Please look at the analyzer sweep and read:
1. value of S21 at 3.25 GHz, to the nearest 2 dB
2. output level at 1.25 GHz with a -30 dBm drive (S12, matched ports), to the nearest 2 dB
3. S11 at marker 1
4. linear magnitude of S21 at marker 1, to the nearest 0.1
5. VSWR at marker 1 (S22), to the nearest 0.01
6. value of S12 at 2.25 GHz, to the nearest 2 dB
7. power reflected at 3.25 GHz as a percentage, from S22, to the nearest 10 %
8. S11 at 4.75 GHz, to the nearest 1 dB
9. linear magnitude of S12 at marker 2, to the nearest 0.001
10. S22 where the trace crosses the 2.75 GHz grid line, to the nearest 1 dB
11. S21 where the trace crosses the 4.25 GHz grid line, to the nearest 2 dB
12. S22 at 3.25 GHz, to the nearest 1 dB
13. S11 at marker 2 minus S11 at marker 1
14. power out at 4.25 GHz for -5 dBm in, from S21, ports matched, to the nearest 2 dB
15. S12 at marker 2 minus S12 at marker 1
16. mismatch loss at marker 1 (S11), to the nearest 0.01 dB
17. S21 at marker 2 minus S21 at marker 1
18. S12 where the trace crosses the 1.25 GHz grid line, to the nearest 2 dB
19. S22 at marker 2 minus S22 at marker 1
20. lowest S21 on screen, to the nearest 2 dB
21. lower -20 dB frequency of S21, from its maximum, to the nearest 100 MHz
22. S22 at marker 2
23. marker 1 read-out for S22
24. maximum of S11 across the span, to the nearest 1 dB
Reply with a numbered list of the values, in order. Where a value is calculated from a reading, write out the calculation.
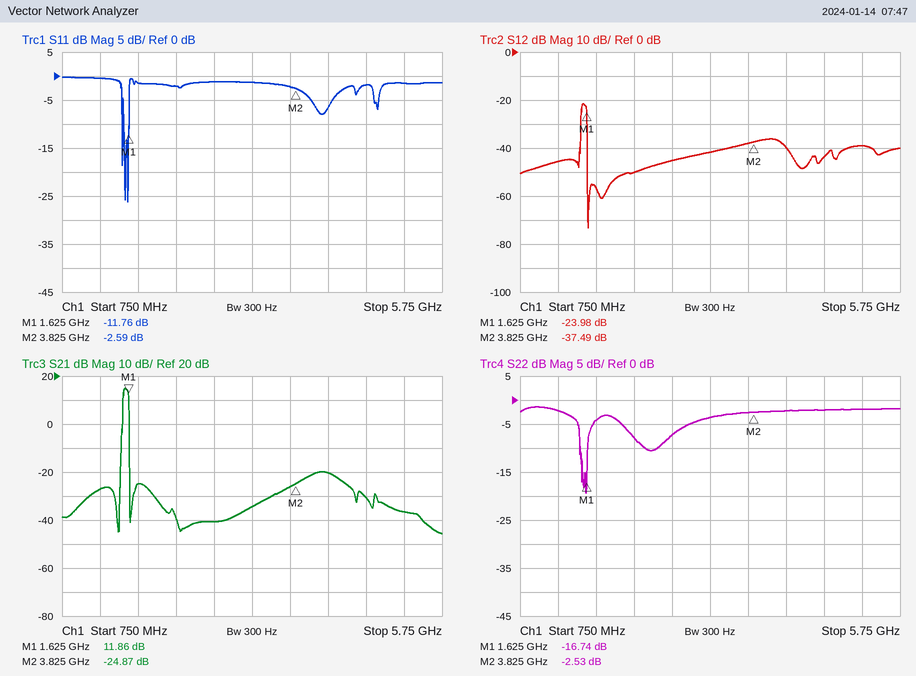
1. -34 dB
2. -30 dBm + (-46 dB) = -76 dBm
3. -11.76 dB
4. 10^(11.86/20) ≈ 3.9
5. (1 + 0.1455)/(1 − 0.1455) ≈ 1.34
6. -50 dB
7. 10^(-4/10) ≈ 40 %
8. -2 dB
9. 10^(-37.49/20) ≈ 0.013
10. -7 dB
11. -20 dB
12. -4 dB
13. -2.59 − (-11.76) = 9.17 dB
14. -5 dBm + (-20 dB) = -26 dBm
15. -37.49 − (-23.98) = -13.51 dB
16. −10 log10(1 − 10^(-11.76/10)) ≈ 0.30 dB
17. -24.87 − (11.86) = -36.73 dB
18. -46 dB
19. -2.53 − (-16.74) = 14.21 dB
20. -46 dB
21. 1.5 GHz
22. -2.53 dB
23. -16.74 dB
24. 0 dB
